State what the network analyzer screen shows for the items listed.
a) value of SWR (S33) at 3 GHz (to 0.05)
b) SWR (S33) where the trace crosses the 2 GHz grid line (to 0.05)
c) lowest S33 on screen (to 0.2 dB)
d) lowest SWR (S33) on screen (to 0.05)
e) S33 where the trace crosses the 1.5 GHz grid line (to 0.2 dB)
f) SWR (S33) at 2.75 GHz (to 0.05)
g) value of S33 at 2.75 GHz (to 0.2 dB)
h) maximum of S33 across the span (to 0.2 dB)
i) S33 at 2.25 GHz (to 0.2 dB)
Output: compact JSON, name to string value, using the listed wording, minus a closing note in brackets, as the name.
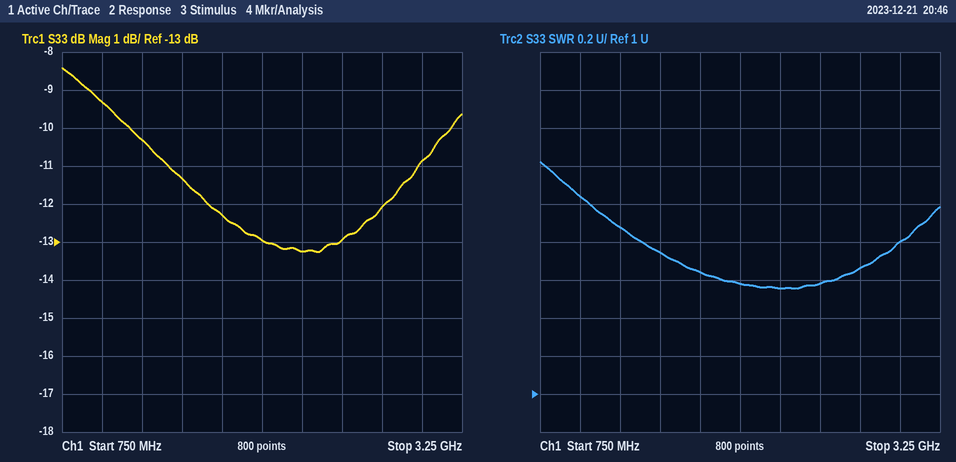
{"value of SWR (S33) at 3 GHz": "1.80", "SWR (S33) where the trace crosses the 2 GHz grid line": "1.60", "lowest S33 on screen": "-13.2 dB", "lowest SWR (S33) on screen": "1.55", "S33 where the trace crosses the 1.5 GHz grid line": "-11.4 dB", "SWR (S33) at 2.75 GHz": "1.65", "value of S33 at 2.75 GHz": "-12.0 dB", "maximum of S33 across the span": "-8.4 dB", "S33 at 2.25 GHz": "-13.2 dB"}
